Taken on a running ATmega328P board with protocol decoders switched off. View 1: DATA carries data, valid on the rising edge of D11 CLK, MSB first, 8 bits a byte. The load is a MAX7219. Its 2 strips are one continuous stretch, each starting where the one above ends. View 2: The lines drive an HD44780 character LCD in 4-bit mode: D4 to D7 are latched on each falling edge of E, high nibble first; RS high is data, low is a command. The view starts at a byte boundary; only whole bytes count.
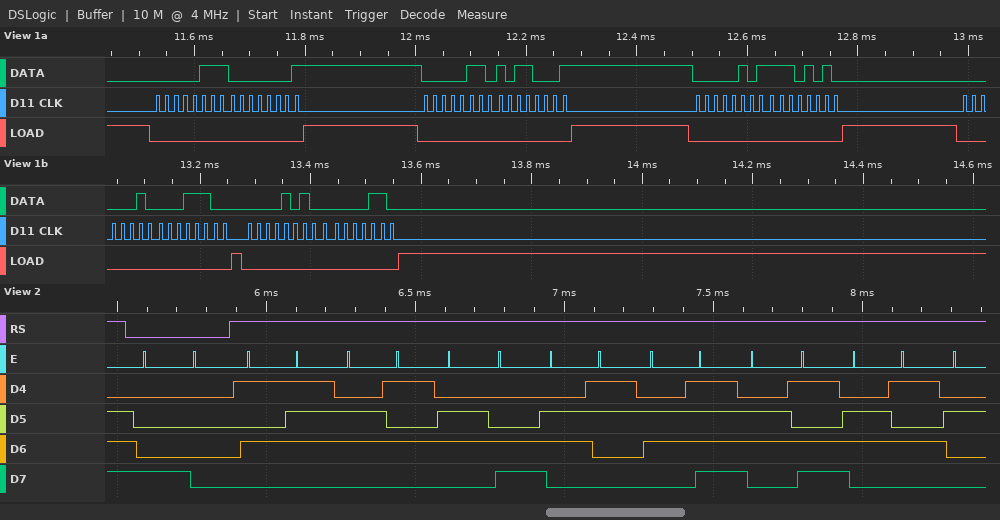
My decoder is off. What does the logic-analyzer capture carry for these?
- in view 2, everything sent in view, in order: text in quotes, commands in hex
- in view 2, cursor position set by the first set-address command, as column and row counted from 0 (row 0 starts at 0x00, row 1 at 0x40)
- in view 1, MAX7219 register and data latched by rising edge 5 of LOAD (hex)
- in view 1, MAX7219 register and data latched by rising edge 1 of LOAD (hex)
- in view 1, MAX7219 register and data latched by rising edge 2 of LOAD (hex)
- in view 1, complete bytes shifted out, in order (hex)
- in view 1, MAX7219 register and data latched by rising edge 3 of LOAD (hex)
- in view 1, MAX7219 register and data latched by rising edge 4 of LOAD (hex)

0x80 "Welcome"
column 0, row 0
register 0xA, data 0x06
register 0x7, data 0x01
register 0x6, data 0xB1
07 01 06 B1 05 EA 02 1C 0A 06
register 0x5, data 0xEA
register 0x2, data 0x1C
